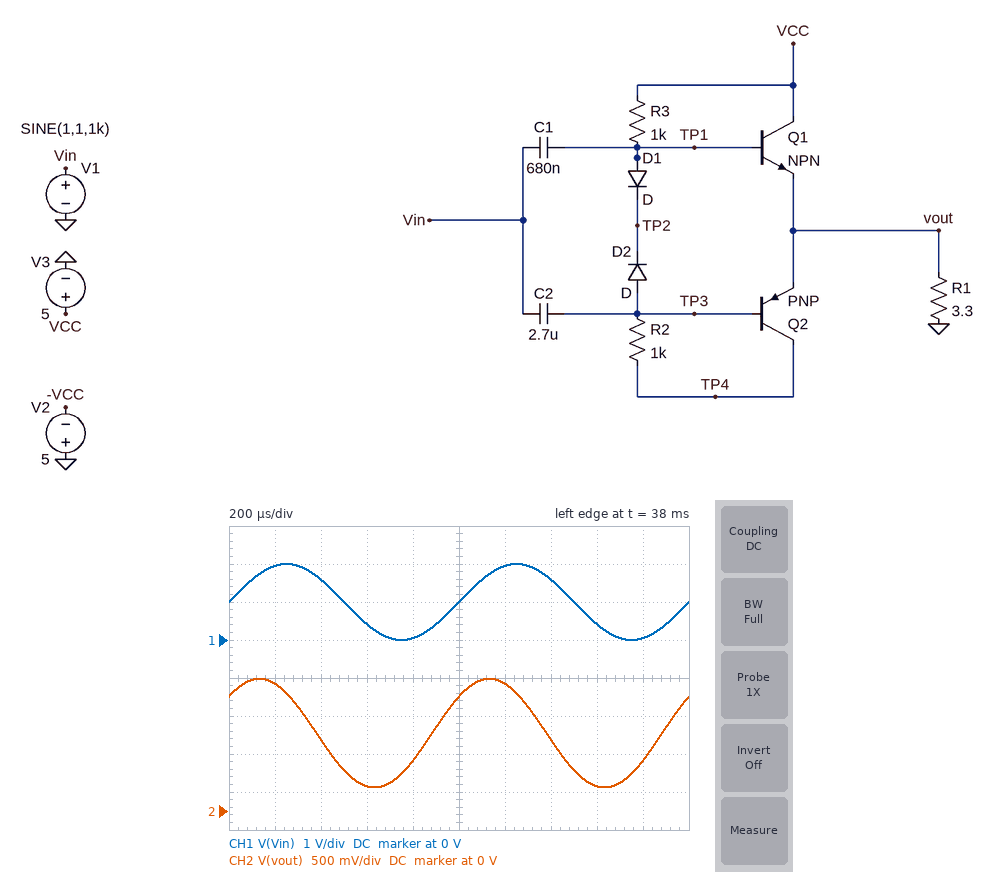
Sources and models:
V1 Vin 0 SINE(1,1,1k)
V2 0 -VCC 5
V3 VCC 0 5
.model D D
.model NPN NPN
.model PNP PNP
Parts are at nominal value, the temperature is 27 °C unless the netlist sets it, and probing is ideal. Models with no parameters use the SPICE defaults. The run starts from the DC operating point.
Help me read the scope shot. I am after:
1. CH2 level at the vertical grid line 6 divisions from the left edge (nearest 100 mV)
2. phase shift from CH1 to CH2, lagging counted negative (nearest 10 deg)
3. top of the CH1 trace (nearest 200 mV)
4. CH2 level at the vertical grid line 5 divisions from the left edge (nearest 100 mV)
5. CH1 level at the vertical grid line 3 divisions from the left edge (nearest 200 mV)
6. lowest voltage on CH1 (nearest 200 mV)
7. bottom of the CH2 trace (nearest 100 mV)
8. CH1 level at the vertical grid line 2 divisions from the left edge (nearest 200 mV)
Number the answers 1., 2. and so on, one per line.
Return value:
1. 1.7 V
2. 40 deg
3. 2.0 V
4. 1.5 V
5. 400 mV
6. 0 V
7. 300 mV
8. 1.6 V
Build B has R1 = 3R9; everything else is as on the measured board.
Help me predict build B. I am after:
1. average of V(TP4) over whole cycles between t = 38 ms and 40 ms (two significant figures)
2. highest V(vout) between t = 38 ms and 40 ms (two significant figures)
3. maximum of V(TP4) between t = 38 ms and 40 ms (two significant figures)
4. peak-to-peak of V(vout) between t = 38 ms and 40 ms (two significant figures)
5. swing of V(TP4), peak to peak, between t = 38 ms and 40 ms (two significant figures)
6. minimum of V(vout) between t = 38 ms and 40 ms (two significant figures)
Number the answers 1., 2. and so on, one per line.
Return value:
1. 1.1 V
2. 1.9 V
3. 2.1 V
4. 1.5 V
5. 2.0 V
6. 400 mV
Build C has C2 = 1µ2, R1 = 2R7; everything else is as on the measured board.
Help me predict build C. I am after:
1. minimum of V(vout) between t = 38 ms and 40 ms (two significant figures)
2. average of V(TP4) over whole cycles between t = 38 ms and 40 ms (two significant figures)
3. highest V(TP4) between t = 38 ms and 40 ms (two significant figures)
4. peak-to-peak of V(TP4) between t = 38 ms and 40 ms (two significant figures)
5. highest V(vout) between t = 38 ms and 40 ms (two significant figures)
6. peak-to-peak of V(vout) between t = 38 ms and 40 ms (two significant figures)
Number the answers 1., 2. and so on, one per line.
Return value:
1. 220 mV
2. 940 mV
3. 1.9 V
4. 2.0 V
5. 1.5 V
6. 1.3 V
